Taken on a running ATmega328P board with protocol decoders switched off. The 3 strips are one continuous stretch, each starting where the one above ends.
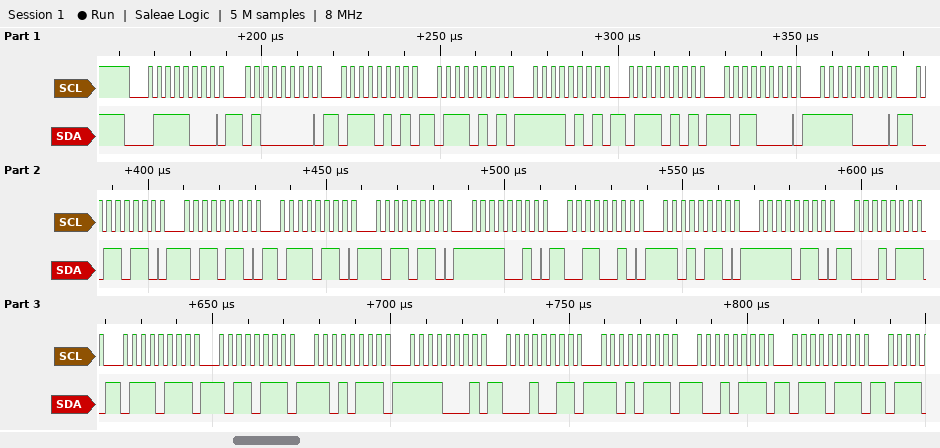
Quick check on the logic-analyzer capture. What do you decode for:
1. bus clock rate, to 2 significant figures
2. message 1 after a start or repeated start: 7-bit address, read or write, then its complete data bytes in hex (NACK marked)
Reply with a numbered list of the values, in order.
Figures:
1. 400 kHz
2. 0x3C write: 40 75 75 F5 75 B0 F0 36 B6 76 B6 F2 32 D6 F6 17 77 B7 D7 F1 13 D7 97 77
